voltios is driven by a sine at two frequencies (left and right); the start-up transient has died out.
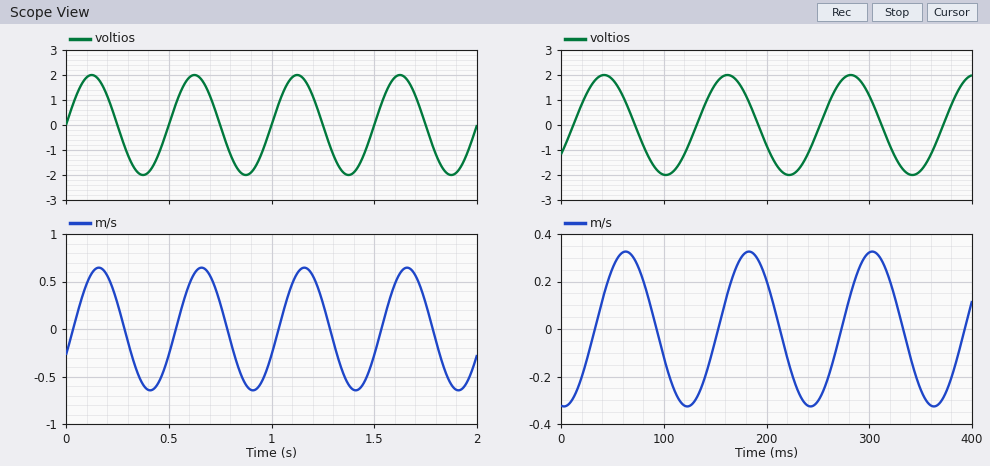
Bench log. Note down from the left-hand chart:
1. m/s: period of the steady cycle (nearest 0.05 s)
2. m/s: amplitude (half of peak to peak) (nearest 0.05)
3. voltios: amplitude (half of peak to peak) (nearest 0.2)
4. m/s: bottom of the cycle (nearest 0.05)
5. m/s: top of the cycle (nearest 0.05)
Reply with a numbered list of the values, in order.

1. 0.50 s
2. 0.65
3. 2.0
4. -0.65
5. 0.65
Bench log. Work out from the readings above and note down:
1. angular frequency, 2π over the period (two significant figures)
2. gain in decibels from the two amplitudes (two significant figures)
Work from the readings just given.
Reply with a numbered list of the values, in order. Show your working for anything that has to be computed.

1. 2π / 0.5 = 13 rad/s
2. 20 log10(0.65 / 2) = -9.8 dB
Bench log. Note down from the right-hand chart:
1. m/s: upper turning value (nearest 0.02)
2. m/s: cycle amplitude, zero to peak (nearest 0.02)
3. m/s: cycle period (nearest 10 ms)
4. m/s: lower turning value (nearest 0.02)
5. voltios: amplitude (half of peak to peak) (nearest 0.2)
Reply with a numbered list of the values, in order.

1. 0.32
2. 0.32
3. 120 ms
4. -0.32
5. 2.0
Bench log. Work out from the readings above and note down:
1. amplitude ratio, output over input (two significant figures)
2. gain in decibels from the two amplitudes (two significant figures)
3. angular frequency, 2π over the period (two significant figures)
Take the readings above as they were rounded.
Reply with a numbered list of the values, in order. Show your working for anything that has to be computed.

1. 0.32 / 2 = 0.16
2. 20 log10(0.32 / 2) = -16 dB
3. 2π / 120 = 0.052 rad/ms
